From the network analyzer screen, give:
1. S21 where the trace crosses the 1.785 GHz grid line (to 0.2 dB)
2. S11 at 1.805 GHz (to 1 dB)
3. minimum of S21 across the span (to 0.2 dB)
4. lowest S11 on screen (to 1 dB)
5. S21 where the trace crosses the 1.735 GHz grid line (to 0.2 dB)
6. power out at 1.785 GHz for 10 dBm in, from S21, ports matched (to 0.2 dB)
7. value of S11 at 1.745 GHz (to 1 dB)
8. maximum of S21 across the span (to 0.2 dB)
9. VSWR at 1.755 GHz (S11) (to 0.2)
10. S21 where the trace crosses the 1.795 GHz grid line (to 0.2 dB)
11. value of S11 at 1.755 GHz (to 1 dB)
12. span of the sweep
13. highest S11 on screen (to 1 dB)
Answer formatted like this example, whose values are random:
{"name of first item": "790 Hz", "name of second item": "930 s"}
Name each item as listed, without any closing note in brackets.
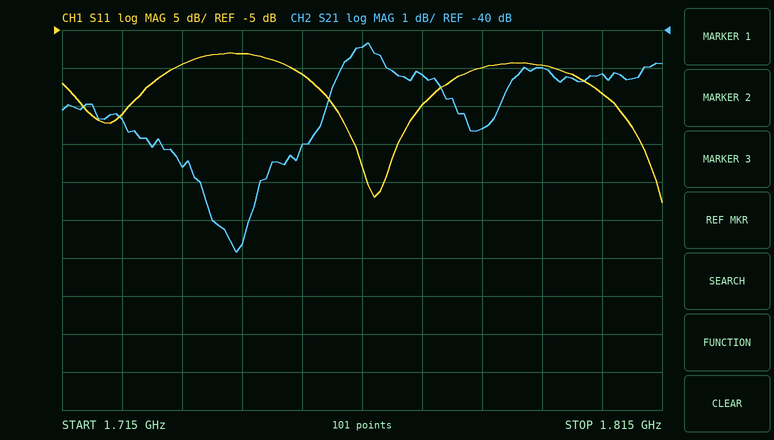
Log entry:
{"S21 where the trace crosses the 1.785 GHz grid line": "-42.6 dB", "S11 at 1.805 GHz": "-13 dB", "minimum of S21 across the span": "-45.8 dB", "lowest S11 on screen": "-28 dB", "S21 where the trace crosses the 1.735 GHz grid line": "-43.6 dB", "power out at 1.785 GHz for 10 dBm in, from S21, ports matched": "-32.6 dBm", "value of S11 at 1.745 GHz": "-8 dB", "maximum of S21 across the span": "-40.4 dB", "VSWR at 1.755 GHz (S11)": "1.8", "S21 where the trace crosses the 1.795 GHz grid line": "-41.0 dB", "value of S11 at 1.755 GHz": "-11 dB", "span of the sweep": "100 MHz", "highest S11 on screen": "-8 dB"}
